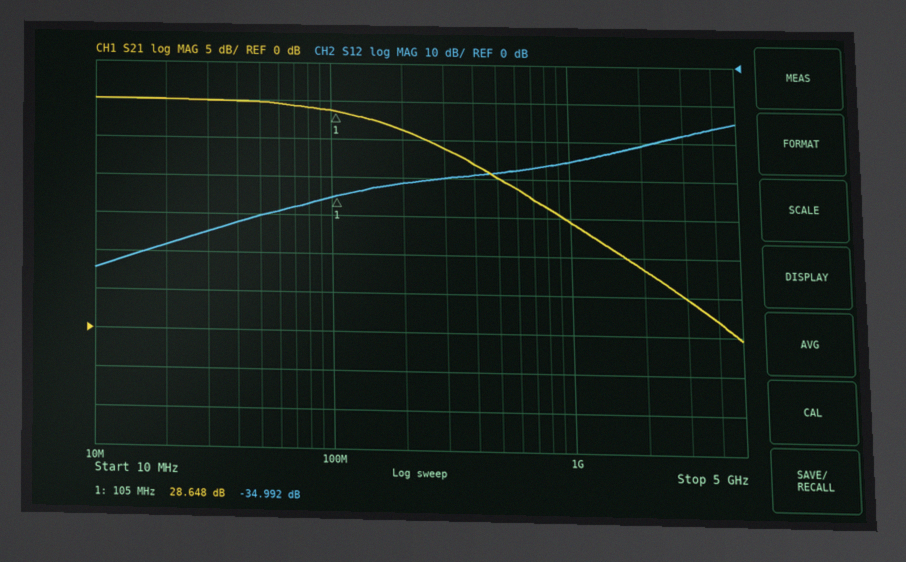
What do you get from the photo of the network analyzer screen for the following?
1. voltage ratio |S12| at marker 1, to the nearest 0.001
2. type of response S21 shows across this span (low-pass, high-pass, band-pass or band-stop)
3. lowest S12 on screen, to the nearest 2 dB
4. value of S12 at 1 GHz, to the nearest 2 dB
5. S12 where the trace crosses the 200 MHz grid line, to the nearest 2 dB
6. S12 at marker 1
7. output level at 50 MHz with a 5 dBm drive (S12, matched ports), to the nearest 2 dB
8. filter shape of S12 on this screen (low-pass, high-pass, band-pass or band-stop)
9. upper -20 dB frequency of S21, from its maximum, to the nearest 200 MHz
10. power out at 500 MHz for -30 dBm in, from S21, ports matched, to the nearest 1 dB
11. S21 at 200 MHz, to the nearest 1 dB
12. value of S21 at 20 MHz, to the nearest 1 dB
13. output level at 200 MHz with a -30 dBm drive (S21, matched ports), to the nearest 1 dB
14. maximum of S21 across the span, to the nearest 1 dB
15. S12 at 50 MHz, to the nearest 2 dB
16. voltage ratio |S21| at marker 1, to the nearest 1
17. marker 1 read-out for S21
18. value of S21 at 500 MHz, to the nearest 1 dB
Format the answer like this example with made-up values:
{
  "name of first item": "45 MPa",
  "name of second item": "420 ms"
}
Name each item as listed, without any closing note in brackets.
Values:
{
  "voltage ratio |S12| at marker 1, to the nearest 0.001": "0.018",
  "type of response S21 shows across this span": "low-pass",
  "lowest S12 on screen, to the nearest 2 dB": "-54 dB",
  "value of S12 at 1 GHz, to the nearest 2 dB": "-26 dB",
  "S12 where the trace crosses the 200 MHz grid line, to the nearest 2 dB": "-32 dB",
  "S12 at marker 1": "-34.992 dB",
  "output level at 50 MHz with a 5 dBm drive (S12, matched ports), to the nearest 2 dB": "-36 dBm",
  "filter shape of S12 on this screen": "high-pass",
  "upper -20 dB frequency of S21, from its maximum, to the nearest 200 MHz": "1.6 GHz",
  "power out at 500 MHz for -30 dBm in, from S21, ports matched, to the nearest 1 dB": "-10 dBm",
  "S21 at 200 MHz, to the nearest 1 dB": "26 dB",
  "value of S21 at 20 MHz, to the nearest 1 dB": "30 dB",
  "output level at 200 MHz with a -30 dBm drive (S21, matched ports), to the nearest 1 dB": "-4 dBm",
  "maximum of S21 across the span, to the nearest 1 dB": "30 dB",
  "S12 at 50 MHz, to the nearest 2 dB": "-40 dB",
  "voltage ratio |S21| at marker 1, to the nearest 1": "27",
  "marker 1 read-out for S21": "28.648 dB",
  "value of S21 at 500 MHz, to the nearest 1 dB": "20 dB"
}
